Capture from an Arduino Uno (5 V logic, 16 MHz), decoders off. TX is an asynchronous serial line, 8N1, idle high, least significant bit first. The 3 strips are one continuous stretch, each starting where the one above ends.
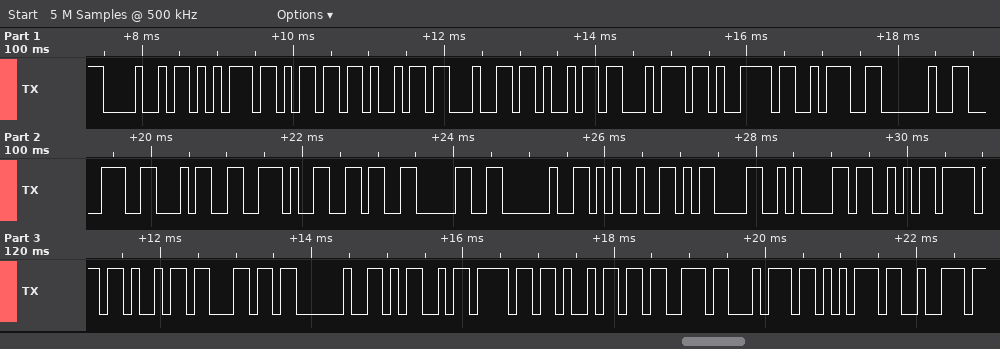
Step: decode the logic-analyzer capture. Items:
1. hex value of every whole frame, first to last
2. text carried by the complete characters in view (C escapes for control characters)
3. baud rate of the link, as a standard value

48 75 6D 69 64 69 74 79 3A 20 38 34 2E 36 30 20 25 0D 0A 53 6F 69 6C 20 4D 6F 69 73 74 75 72
"Humidity: 84.60 %\r\nSoil Moistur"
9600 baud
